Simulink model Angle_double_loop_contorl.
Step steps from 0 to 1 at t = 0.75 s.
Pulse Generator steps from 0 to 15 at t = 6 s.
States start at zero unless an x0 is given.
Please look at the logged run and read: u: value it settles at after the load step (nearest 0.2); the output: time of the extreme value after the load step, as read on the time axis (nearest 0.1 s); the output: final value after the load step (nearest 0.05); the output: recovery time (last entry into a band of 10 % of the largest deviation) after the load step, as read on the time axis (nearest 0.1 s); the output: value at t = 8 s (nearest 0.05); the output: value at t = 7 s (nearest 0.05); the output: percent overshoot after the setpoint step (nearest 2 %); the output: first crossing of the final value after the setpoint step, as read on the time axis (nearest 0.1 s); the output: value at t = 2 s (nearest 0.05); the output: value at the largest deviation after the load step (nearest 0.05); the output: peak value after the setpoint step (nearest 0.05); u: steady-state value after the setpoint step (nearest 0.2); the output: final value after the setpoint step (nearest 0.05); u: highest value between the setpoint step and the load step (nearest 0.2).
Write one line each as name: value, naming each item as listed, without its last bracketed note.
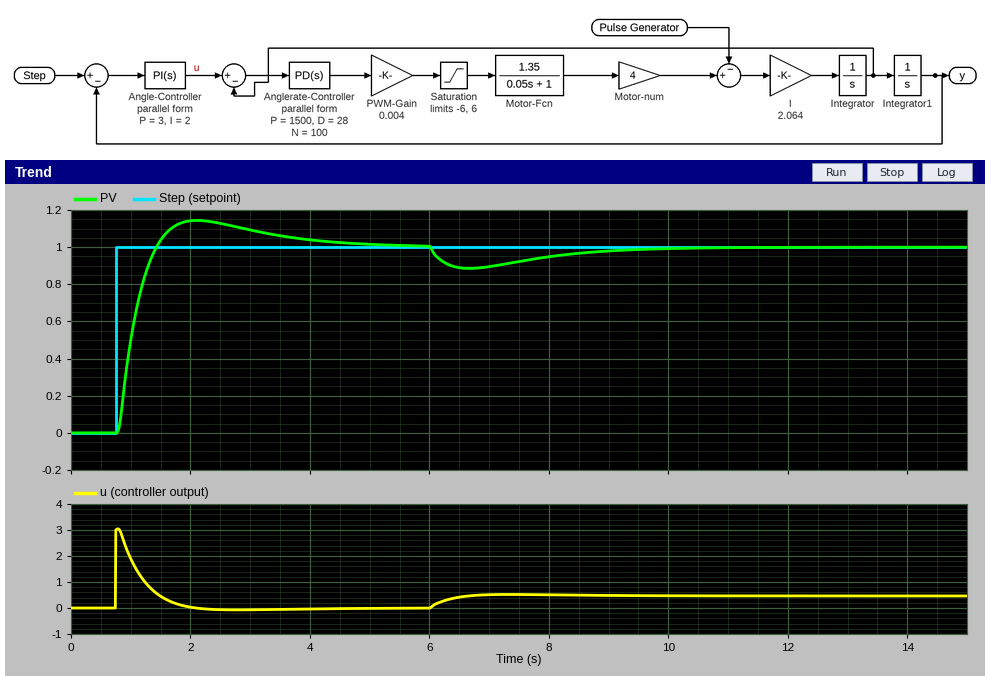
u: value it settles at after the load step: 0.4
the output: time of the extreme value after the load step, as read on the time axis: 6.7 s
the output: final value after the load step: 1.00
the output: recovery time (last entry into a band of 10 % of the largest deviation) after the load step, as read on the time axis: 9.6 s
the output: value at t = 8 s: 0.95
the output: value at t = 7 s: 0.90
the output: percent overshoot after the setpoint step: 14 %
the output: first crossing of the final value after the setpoint step, as read on the time axis: 1.4 s
the output: value at t = 2 s: 1.15
the output: value at the largest deviation after the load step: 0.90
the output: peak value after the setpoint step: 1.15
u: steady-state value after the setpoint step: 0.0
the output: final value after the setpoint step: 1.00
u: highest value between the setpoint step and the load step: 3.0
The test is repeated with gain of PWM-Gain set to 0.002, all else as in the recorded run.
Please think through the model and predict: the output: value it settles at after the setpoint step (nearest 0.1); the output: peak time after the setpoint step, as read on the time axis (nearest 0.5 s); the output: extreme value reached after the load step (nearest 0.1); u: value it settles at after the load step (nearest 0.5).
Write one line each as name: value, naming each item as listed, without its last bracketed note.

the output: value it settles at after the setpoint step: 1.0
the output: peak time after the setpoint step, as read on the time axis: 2.0 s
the output: extreme value reached after the load step: 0.8
u: value it settles at after the load step: 1.0
